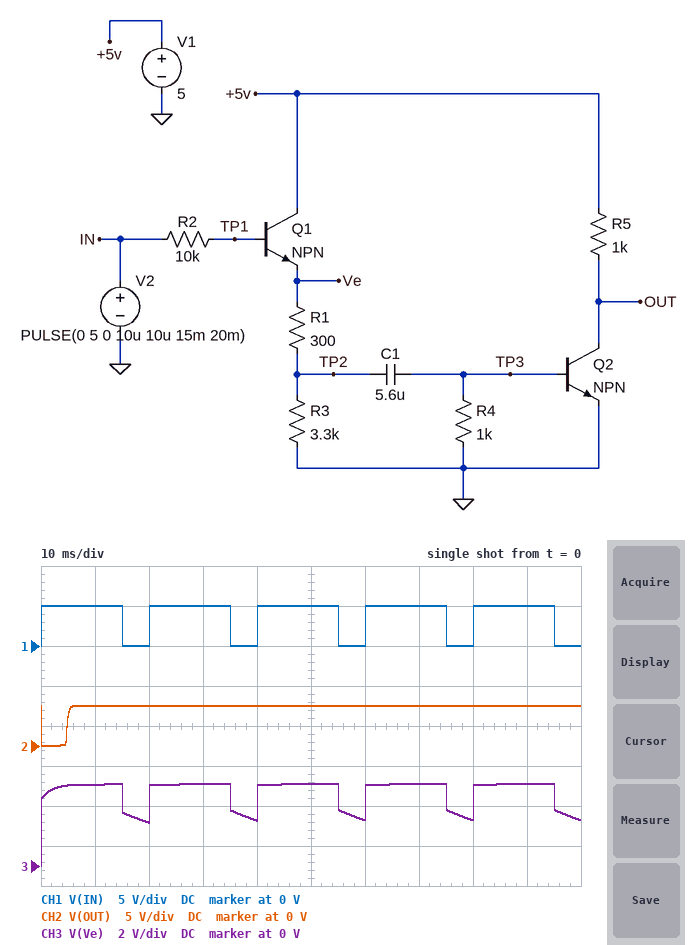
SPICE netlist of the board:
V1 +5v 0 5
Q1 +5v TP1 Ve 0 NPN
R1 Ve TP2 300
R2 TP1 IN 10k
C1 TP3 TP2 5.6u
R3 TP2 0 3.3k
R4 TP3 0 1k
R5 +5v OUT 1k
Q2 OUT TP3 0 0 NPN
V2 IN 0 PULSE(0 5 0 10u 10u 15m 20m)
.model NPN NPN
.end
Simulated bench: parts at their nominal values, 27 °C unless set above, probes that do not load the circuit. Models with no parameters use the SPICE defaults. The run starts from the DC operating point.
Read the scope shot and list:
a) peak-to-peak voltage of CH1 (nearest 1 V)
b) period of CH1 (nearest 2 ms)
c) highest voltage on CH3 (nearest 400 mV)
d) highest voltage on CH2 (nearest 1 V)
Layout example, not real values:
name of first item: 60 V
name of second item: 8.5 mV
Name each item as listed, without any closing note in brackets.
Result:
peak-to-peak voltage of CH1: 5 V
period of CH1: 20 ms
highest voltage on CH3: 4.0 V
highest voltage on CH2: 5 V
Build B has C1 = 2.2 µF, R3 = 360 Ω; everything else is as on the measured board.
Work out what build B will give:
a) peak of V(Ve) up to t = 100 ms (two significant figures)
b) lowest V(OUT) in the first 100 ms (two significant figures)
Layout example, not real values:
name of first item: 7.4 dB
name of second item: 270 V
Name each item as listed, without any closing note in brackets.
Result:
peak of V(Ve) up to t = 100 ms: 3.6 V
lowest V(OUT) in the first 100 ms: 28 mV
